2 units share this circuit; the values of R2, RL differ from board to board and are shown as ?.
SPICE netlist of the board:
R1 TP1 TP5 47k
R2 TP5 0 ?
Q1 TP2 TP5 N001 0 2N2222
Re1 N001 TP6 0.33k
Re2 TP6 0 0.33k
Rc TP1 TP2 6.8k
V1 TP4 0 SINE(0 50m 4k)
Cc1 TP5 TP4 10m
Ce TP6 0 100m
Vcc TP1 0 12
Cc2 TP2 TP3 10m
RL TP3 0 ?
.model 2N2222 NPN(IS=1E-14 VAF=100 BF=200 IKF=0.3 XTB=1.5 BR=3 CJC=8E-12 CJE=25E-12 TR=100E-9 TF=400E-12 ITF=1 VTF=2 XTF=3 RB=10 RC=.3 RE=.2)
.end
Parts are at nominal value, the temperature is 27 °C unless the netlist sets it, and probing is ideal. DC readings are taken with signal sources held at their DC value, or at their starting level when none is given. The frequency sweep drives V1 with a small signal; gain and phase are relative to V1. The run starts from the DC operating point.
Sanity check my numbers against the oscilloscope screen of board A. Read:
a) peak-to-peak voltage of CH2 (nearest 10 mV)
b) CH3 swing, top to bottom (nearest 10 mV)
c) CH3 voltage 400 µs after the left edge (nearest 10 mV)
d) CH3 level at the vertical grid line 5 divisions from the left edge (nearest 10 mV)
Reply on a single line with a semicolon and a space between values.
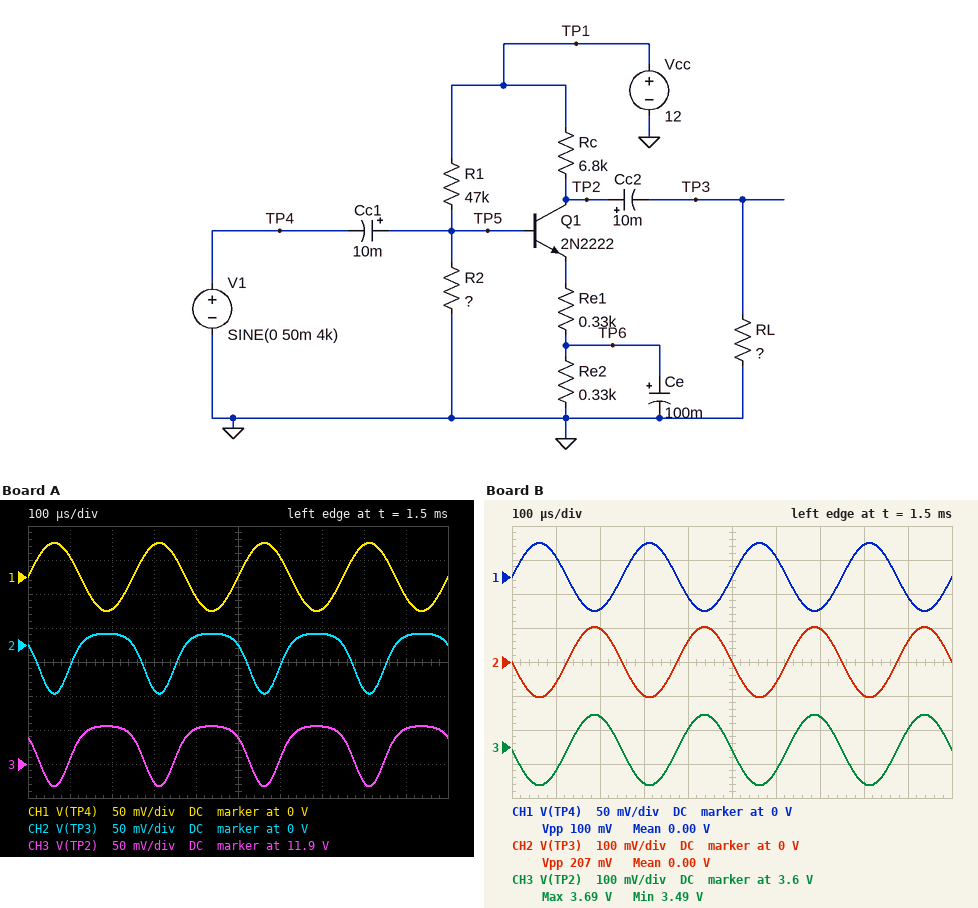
90 mV; 90 mV; 11.95 V; 11.94 V
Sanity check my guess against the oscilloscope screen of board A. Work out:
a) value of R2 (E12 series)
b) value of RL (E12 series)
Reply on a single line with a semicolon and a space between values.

2.2 kΩ; 3.3 kΩ
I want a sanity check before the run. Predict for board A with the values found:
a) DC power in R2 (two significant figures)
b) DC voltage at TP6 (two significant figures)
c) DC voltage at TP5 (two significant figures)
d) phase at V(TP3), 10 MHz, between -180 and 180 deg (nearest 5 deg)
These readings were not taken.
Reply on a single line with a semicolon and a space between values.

130 µW; 3.0 mV; 540 mV; 95 deg
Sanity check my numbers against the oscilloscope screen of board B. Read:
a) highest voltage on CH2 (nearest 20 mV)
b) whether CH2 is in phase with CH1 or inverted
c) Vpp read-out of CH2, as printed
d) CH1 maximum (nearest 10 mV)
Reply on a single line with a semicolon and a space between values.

100 mV; inverted; 207 mV; 50 mV
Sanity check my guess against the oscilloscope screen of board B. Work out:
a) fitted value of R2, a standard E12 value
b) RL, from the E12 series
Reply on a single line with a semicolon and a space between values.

6.8 kΩ; 820 Ω
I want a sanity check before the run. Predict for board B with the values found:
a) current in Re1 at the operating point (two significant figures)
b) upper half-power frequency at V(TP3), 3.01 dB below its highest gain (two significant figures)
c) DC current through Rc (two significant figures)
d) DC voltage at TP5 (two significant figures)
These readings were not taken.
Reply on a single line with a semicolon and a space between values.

1.2 mA; 74 MHz; 1.2 mA; 1.5 V
